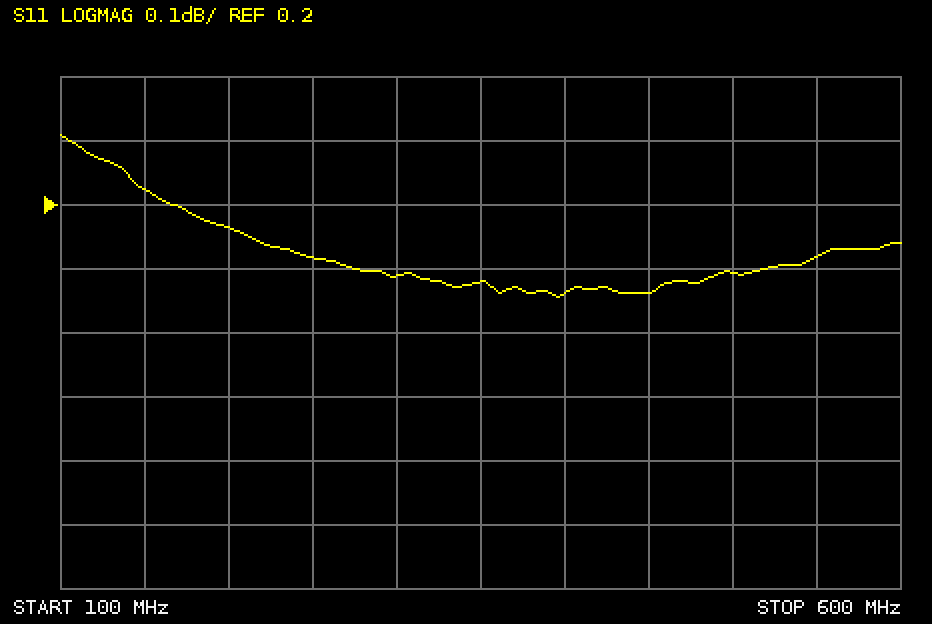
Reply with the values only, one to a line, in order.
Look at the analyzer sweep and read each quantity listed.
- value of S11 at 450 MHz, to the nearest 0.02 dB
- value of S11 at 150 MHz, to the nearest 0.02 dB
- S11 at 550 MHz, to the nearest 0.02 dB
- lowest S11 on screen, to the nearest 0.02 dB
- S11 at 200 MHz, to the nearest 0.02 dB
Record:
0.06 dB
0.22 dB
0.12 dB
0.06 dB
0.16 dB
